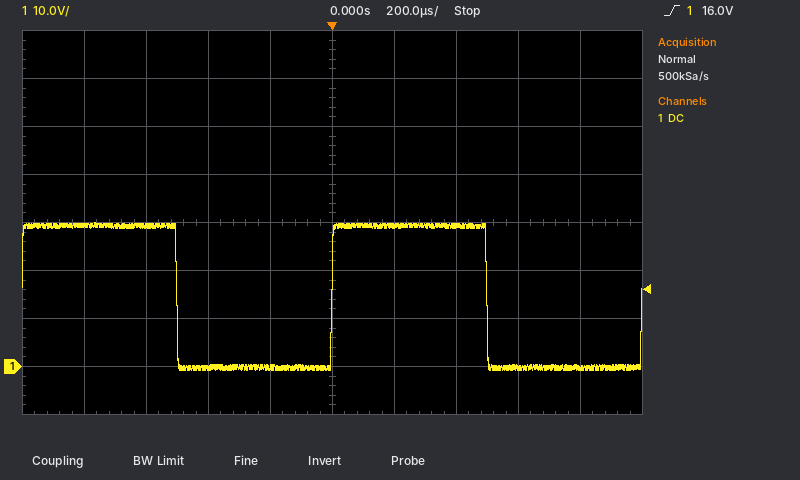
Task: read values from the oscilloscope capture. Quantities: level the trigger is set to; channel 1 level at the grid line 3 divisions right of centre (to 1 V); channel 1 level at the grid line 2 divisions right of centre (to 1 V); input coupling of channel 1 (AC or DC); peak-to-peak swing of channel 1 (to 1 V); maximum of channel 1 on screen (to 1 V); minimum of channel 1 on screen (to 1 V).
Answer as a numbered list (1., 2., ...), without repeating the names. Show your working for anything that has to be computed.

1. 16.0 V
2. 0 V
3. 29 V
4. DC
5. 30 V − (-1 V) = 31 V
6. 30 V
7. -1 V
